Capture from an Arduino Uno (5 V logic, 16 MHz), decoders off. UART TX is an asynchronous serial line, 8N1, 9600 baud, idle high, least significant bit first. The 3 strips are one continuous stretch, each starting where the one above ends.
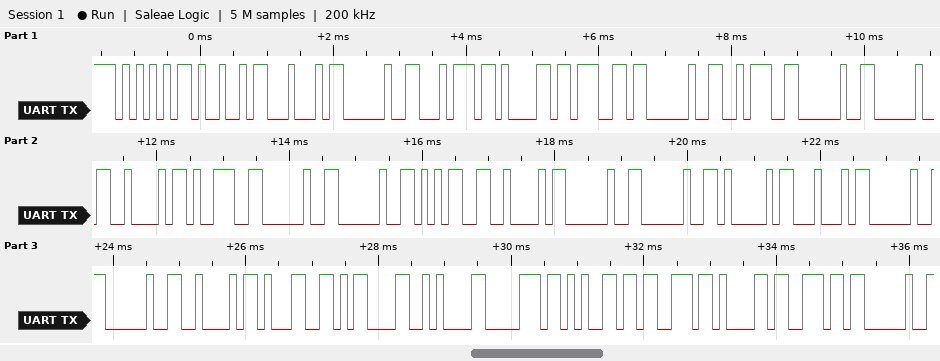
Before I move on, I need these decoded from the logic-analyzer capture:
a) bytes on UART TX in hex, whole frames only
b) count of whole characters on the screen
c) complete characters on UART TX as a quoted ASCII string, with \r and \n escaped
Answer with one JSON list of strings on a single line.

["0x55 0x49 0x44 0x20 0x74 0x61 0x67 0x20 0x3A 0x20 0x20 0x42 0x39 0x20 0x20 0x35 0x42 0x20 0x20 0x41 0x44 0x20 0x20 0x42 0x31 0x0D 0x0A 0x70 0x65 0x73 0x61 0x6E 0x20", "33", "\"UID tag :  B9  5B  AD  B1\\r\\npesan \""]
